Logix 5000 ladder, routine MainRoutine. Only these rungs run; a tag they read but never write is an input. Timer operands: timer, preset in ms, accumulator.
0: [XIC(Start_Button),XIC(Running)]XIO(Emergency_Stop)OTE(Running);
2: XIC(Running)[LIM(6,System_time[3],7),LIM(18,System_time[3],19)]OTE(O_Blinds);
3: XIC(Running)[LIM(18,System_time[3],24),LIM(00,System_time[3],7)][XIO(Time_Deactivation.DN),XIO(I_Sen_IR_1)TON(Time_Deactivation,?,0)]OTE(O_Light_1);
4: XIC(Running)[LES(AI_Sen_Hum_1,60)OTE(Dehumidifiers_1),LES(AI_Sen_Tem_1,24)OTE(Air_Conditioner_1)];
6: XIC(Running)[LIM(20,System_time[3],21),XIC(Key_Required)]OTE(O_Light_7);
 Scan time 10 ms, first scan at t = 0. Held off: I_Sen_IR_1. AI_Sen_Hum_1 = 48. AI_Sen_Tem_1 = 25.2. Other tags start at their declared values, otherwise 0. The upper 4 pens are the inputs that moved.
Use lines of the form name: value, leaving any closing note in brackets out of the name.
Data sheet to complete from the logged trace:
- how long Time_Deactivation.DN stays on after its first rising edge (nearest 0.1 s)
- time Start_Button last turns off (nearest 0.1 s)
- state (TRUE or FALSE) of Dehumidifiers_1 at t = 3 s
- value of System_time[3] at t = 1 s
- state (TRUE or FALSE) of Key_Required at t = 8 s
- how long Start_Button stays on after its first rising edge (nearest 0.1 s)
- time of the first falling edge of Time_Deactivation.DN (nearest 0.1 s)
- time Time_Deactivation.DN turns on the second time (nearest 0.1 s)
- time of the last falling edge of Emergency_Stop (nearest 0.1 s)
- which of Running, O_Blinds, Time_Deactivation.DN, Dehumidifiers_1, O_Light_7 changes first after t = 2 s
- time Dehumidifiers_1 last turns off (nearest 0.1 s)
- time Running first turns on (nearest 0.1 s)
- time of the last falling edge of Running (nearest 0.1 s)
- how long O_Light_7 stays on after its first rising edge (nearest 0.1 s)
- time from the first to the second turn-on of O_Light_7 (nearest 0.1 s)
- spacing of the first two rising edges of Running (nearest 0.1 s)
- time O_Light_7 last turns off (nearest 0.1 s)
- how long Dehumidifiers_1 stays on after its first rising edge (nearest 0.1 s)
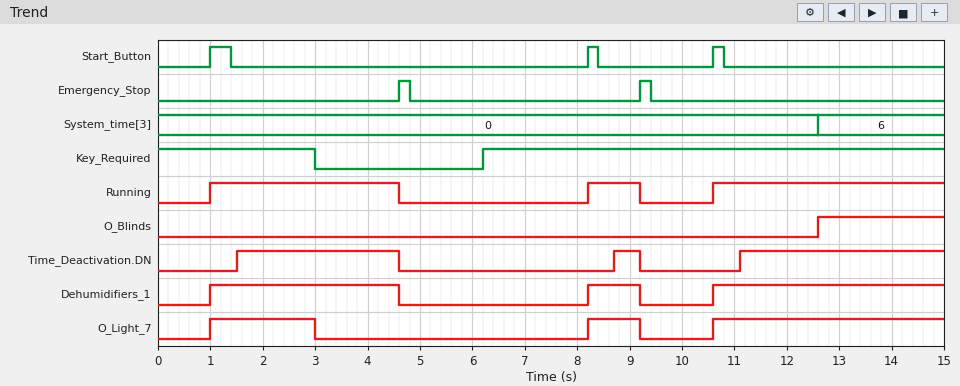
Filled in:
how long Time_Deactivation.DN stays on after its first rising edge: 3.1 s
time Start_Button last turns off: 10.8 s
state (TRUE or FALSE) of Dehumidifiers_1 at t = 3 s: TRUE
value of System_time[3] at t = 1 s: 0
state (TRUE or FALSE) of Key_Required at t = 8 s: TRUE
how long Start_Button stays on after its first rising edge: 0.4 s
time of the first falling edge of Time_Deactivation.DN: 4.6 s
time Time_Deactivation.DN turns on the second time: 8.7 s
time of the last falling edge of Emergency_Stop: 9.4 s
which of Running, O_Blinds, Time_Deactivation.DN, Dehumidifiers_1, O_Light_7 changes first after t = 2 s: O_Light_7
time Dehumidifiers_1 last turns off: 9.2 s
time Running first turns on: 1.0 s
time of the last falling edge of Running: 9.2 s
how long O_Light_7 stays on after its first rising edge: 2.0 s
time from the first to the second turn-on of O_Light_7: 7.2 s
spacing of the first two rising edges of Running: 7.2 s
time O_Light_7 last turns off: 9.2 s
how long Dehumidifiers_1 stays on after its first rising edge: 3.6 s
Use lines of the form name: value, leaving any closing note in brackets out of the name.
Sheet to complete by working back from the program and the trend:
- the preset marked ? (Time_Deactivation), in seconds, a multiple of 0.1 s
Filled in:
the preset marked ? (Time_Deactivation), in seconds, a multiple of 0.1 s: 0.5 s
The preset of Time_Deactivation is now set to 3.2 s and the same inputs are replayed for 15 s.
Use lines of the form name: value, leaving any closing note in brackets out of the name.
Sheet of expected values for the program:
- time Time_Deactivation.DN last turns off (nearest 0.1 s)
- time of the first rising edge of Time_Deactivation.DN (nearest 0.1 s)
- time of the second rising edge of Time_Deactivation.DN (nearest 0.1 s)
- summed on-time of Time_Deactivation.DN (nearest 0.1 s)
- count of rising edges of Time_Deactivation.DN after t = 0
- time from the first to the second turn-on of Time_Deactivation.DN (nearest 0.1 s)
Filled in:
time Time_Deactivation.DN last turns off: 4.6 s
time of the first rising edge of Time_Deactivation.DN: 4.2 s
time of the second rising edge of Time_Deactivation.DN: 13.8 s
summed on-time of Time_Deactivation.DN: 1.6 s
count of rising edges of Time_Deactivation.DN after t = 0: 2
time from the first to the second turn-on of Time_Deactivation.DN: 9.6 s
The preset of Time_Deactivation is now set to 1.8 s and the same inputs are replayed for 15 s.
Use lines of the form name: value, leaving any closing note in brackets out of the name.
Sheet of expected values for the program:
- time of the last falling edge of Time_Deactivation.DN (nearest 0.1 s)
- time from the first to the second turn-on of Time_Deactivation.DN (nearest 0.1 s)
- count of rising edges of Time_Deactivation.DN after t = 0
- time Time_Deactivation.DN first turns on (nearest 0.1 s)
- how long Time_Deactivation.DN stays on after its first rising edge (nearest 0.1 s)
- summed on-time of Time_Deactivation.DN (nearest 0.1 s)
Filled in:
time of the last falling edge of Time_Deactivation.DN: 4.6 s
time from the first to the second turn-on of Time_Deactivation.DN: 9.6 s
count of rising edges of Time_Deactivation.DN after t = 0: 2
time Time_Deactivation.DN first turns on: 2.8 s
how long Time_Deactivation.DN stays on after its first rising edge: 1.8 s
summed on-time of Time_Deactivation.DN: 4.4 s
